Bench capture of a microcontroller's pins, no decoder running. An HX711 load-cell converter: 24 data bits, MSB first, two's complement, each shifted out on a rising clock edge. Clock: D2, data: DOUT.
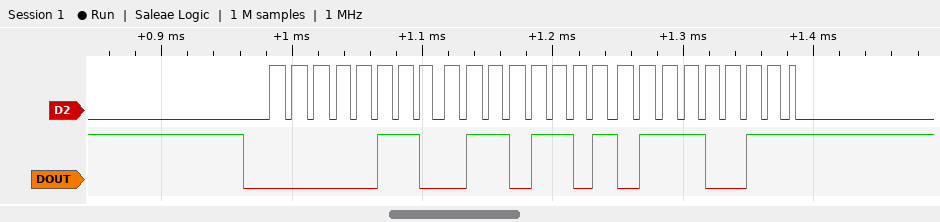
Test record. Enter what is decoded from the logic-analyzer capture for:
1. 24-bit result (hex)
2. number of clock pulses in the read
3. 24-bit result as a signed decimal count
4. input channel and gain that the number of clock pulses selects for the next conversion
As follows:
0x066D73
25
421235
channel A, gain 128
